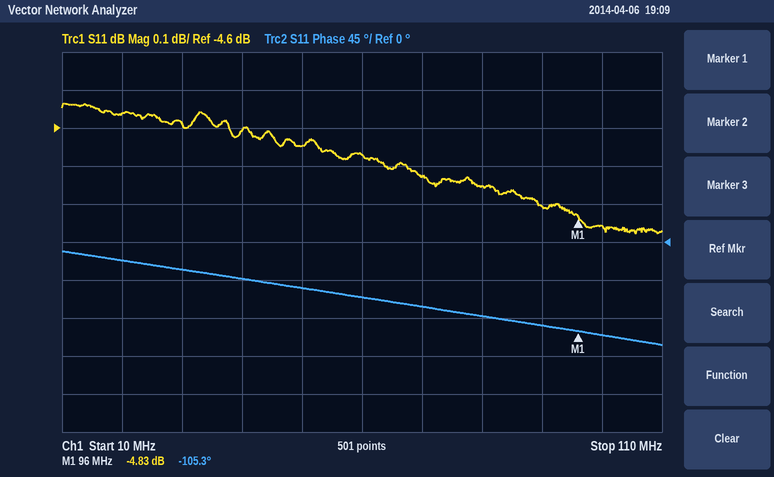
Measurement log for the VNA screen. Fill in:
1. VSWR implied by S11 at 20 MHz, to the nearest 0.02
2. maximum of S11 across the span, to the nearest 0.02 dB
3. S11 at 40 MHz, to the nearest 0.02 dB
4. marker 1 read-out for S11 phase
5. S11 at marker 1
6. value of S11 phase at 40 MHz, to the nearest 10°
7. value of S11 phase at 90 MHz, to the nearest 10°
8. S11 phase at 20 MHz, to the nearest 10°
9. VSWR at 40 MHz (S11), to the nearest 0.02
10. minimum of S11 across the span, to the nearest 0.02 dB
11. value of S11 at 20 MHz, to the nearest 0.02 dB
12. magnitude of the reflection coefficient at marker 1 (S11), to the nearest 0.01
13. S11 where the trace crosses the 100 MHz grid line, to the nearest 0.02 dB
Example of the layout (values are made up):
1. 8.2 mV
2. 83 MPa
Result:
1. 3.90
2. -4.54 dB
3. -4.60 dB
4. -105.3°
5. -4.83 dB
6. -40°
7. -100°
8. -20°
9. 3.86
10. -4.88 dB
11. -4.56 dB
12. 0.57
13. -4.86 dB
